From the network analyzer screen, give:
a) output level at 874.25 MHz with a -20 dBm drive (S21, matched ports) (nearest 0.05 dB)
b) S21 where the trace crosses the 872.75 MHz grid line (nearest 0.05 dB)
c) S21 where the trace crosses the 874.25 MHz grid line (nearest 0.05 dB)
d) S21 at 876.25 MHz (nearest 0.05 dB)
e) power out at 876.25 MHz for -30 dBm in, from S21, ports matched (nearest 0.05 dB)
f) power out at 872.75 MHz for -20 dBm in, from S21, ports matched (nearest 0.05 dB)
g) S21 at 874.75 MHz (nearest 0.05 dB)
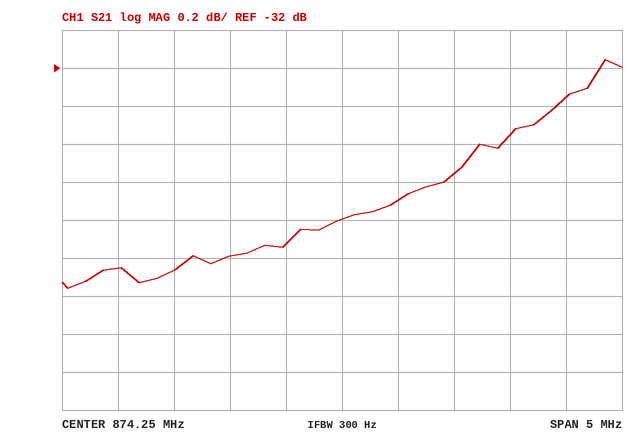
-52.80 dBm
-33.05 dB
-32.80 dB
-32.15 dB
-62.15 dBm
-53.05 dBm
-32.70 dB
